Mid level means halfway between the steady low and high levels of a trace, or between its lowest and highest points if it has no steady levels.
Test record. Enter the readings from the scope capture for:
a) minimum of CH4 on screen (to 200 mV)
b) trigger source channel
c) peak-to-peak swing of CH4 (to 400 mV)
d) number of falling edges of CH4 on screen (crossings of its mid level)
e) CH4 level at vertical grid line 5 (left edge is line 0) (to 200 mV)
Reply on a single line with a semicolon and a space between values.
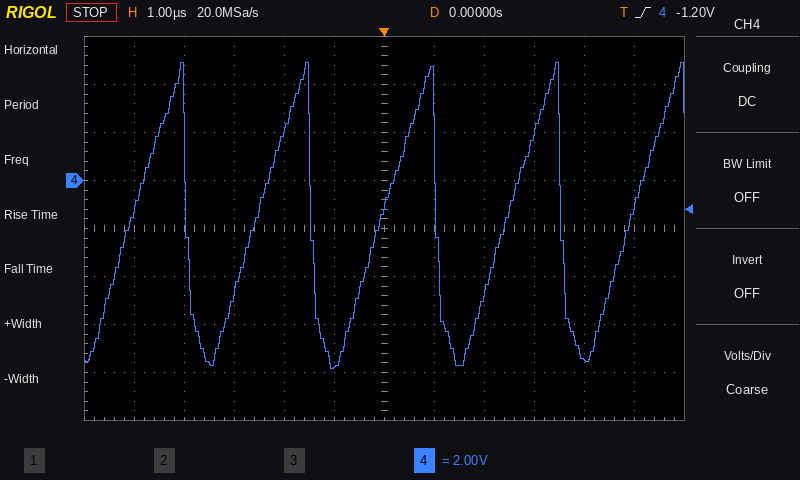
-7.8 V; CH4; 12.8 V; 4; -7.8 V
